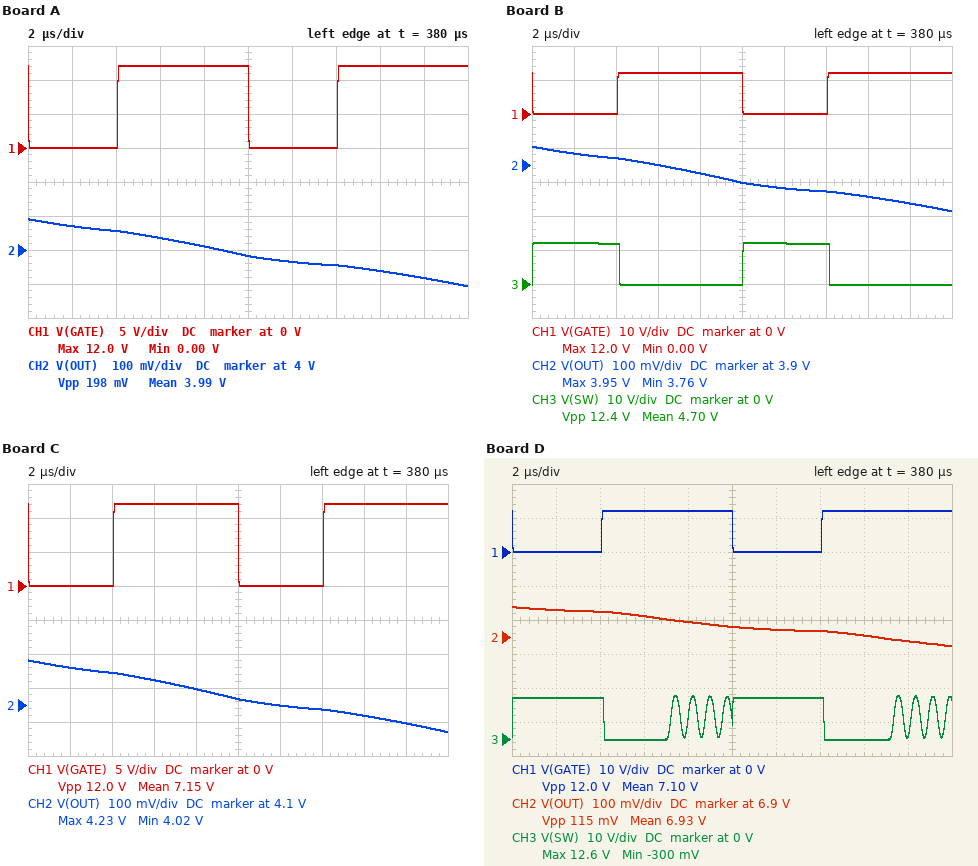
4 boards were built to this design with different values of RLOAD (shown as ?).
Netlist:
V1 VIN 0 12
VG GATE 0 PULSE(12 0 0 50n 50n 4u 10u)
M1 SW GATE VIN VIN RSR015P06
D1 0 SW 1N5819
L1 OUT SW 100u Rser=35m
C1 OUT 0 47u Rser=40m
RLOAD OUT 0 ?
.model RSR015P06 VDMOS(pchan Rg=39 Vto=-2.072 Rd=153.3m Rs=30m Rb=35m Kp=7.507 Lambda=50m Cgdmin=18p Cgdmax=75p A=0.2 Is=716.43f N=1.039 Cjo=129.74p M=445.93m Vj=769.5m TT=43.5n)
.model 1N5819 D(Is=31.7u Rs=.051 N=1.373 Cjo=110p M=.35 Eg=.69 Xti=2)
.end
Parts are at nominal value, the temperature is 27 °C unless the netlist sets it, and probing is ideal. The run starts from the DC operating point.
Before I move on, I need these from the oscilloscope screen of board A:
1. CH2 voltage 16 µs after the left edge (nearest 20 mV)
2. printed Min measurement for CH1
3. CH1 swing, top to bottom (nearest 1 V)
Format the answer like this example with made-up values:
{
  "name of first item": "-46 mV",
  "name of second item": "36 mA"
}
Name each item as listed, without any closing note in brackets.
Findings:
{
  "CH2 voltage 16 µs after the left edge": "3.94 V",
  "printed Min measurement for CH1": "0.00 V",
  "CH1 swing, top to bottom": "12 V"
}
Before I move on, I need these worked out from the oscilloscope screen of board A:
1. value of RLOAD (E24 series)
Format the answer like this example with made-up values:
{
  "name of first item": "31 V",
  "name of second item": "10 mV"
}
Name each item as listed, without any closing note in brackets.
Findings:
{
  "value of RLOAD": "4.7 Ω"
}
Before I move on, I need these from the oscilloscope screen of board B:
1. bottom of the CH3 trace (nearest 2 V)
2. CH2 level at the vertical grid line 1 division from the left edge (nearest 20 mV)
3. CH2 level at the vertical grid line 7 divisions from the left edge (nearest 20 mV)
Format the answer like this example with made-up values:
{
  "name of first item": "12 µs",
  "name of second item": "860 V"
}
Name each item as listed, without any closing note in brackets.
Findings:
{
  "bottom of the CH3 trace": "0 V",
  "CH2 level at the vertical grid line 1 division from the left edge": "3.94 V",
  "CH2 level at the vertical grid line 7 divisions from the left edge": "3.82 V"
}
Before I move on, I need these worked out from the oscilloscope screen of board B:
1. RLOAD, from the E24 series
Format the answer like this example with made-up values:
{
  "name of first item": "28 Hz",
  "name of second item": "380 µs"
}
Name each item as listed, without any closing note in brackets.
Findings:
{
  "RLOAD, from the E24 series": "4.3 Ω"
}
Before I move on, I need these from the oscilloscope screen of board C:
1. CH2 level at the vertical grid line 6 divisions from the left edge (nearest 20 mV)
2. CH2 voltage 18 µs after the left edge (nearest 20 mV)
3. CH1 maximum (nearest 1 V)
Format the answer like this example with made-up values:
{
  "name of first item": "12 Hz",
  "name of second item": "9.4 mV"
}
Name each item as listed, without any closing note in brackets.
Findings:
{
  "CH2 level at the vertical grid line 6 divisions from the left edge": "4.10 V",
  "CH2 voltage 18 µs after the left edge": "4.04 V",
  "CH1 maximum": "12 V"
}
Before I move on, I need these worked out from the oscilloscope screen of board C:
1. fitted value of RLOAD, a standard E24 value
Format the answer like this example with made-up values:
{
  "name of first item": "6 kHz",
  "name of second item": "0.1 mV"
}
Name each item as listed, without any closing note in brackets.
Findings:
{
  "fitted value of RLOAD, a standard E24 value": "5.1 Ω"
}
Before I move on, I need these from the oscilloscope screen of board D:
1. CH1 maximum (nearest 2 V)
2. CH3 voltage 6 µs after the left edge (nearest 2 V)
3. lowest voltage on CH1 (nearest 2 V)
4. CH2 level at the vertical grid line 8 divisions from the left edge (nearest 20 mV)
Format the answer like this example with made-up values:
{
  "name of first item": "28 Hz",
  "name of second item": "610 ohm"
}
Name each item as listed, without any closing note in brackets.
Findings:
{
  "CH1 maximum": "12 V",
  "CH3 voltage 6 µs after the left edge": "0 V",
  "lowest voltage on CH1": "0 V",
  "CH2 level at the vertical grid line 8 divisions from the left edge": "6.90 V"
}
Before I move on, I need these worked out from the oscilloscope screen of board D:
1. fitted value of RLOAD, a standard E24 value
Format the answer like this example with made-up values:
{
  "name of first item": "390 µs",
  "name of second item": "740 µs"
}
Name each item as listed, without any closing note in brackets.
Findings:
{
  "fitted value of RLOAD, a standard E24 value": "20 Ω"
}
